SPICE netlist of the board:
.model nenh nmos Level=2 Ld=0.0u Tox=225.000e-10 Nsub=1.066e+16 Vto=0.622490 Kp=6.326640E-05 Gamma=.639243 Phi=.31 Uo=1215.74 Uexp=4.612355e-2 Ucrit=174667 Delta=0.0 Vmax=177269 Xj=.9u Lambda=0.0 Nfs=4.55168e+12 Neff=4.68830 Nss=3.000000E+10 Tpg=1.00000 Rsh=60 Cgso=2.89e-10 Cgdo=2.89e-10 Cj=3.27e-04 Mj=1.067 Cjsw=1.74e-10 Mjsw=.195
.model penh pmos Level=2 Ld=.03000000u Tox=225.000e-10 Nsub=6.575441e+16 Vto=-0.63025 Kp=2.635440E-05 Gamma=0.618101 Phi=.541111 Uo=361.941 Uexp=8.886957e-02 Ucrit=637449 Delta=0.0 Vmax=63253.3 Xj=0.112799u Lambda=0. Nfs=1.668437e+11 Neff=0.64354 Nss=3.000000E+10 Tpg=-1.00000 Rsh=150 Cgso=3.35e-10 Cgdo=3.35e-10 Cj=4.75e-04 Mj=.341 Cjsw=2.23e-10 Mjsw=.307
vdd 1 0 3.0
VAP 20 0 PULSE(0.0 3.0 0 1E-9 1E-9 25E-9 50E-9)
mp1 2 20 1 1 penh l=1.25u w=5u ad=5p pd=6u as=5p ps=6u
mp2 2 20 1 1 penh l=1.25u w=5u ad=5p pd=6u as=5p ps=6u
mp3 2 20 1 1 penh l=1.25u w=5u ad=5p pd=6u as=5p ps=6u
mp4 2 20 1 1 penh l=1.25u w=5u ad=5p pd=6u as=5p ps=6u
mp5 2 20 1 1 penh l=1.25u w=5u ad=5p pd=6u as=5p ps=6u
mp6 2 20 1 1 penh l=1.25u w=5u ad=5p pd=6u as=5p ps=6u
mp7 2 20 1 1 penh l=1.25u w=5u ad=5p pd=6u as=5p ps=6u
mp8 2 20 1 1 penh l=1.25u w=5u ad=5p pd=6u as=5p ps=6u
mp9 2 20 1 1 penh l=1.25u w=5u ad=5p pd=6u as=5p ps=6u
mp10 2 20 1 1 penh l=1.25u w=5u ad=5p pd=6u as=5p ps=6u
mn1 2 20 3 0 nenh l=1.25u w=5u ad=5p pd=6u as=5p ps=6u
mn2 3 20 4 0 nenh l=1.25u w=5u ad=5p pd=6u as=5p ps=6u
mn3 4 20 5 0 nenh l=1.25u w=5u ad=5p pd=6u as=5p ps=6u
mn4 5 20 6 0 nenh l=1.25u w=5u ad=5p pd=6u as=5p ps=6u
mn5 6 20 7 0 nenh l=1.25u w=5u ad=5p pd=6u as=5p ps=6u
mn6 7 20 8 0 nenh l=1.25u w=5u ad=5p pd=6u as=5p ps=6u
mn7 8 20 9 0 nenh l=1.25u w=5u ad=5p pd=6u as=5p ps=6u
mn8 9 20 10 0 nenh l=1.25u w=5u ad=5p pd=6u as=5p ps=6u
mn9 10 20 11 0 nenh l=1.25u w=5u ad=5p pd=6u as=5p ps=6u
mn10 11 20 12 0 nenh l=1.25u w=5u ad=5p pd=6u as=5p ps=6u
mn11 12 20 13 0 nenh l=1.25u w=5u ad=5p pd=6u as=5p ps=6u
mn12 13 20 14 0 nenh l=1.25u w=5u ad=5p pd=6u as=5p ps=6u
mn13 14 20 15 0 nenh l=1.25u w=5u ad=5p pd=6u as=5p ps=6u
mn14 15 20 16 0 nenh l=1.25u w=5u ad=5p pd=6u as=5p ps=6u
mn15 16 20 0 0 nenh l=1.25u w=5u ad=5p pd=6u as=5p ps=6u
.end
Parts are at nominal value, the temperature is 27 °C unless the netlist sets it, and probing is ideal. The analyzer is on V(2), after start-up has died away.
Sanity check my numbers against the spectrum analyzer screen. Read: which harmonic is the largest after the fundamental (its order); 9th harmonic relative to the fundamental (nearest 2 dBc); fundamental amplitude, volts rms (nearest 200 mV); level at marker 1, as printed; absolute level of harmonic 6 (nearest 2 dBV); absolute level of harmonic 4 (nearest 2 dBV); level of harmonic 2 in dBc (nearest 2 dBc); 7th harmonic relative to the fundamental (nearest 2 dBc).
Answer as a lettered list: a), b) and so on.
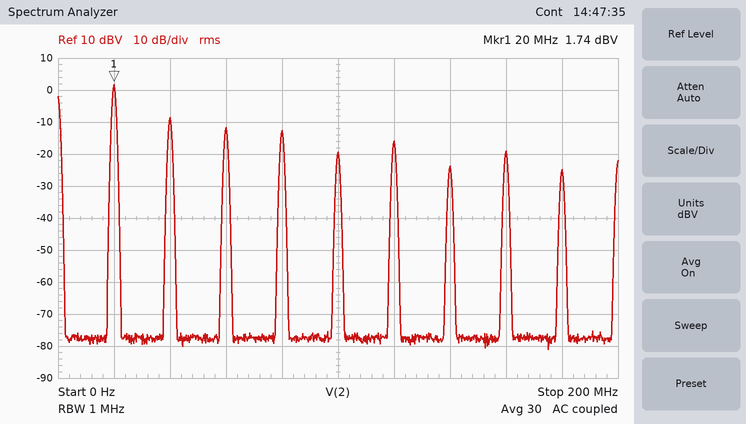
a) 2
b) -26 dBc
c) 1.2 V
d) 1.74 dBV
e) -16 dBV
f) -12 dBV
g) -10 dBc
h) -26 dBc
